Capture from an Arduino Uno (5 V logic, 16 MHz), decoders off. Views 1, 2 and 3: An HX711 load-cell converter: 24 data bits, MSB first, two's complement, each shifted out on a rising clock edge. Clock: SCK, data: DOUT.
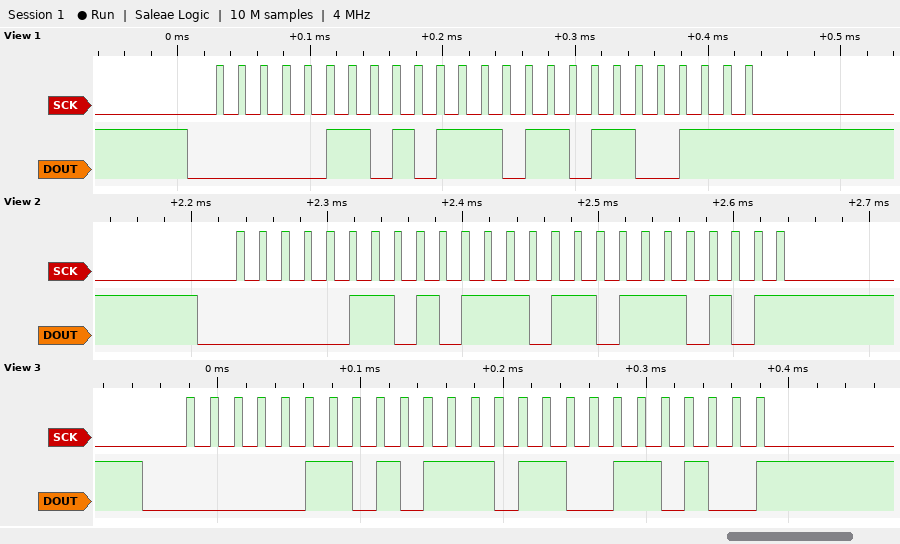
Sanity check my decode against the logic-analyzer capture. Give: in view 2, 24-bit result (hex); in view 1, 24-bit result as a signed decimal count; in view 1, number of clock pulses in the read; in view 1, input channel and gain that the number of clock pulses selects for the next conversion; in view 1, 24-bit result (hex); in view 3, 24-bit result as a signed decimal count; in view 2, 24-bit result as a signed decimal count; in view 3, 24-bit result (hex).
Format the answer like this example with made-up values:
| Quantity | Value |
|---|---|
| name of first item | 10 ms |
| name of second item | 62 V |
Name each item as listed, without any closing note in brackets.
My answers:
| Quantity | Value |
|---|---|
| in view 2, 24-bit result | 0x06BB75 |
| in view 1, 24-bit result as a signed decimal count | 441191 |
| in view 1, number of clock pulses in the read | 25 |
| in view 1, input channel and gain that the number of clock pulses selects for the next conversion | channel A, gain 128 |
| in view 1, 24-bit result | 0x06BB67 |
| in view 3, 24-bit result as a signed decimal count | 441140 |
| in view 2, 24-bit result as a signed decimal count | 441205 |
| in view 3, 24-bit result | 0x06BB34 |
